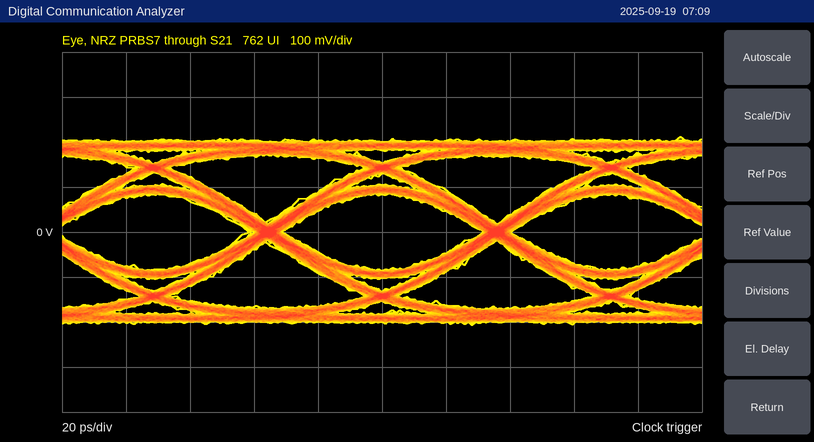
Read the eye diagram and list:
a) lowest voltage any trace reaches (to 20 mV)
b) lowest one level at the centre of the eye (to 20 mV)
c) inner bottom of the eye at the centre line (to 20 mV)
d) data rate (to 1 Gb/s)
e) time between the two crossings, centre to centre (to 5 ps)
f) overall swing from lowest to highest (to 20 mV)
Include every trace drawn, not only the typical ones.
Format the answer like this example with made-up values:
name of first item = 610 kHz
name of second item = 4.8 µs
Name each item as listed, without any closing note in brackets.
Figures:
lowest voltage any trace reaches = -200 mV
lowest one level at the centre of the eye = 80 mV
inner bottom of the eye at the centre line = -80 mV
data rate = 14 Gb/s
time between the two crossings, centre to centre = 70 ps
overall swing from lowest to highest = 420 mV
